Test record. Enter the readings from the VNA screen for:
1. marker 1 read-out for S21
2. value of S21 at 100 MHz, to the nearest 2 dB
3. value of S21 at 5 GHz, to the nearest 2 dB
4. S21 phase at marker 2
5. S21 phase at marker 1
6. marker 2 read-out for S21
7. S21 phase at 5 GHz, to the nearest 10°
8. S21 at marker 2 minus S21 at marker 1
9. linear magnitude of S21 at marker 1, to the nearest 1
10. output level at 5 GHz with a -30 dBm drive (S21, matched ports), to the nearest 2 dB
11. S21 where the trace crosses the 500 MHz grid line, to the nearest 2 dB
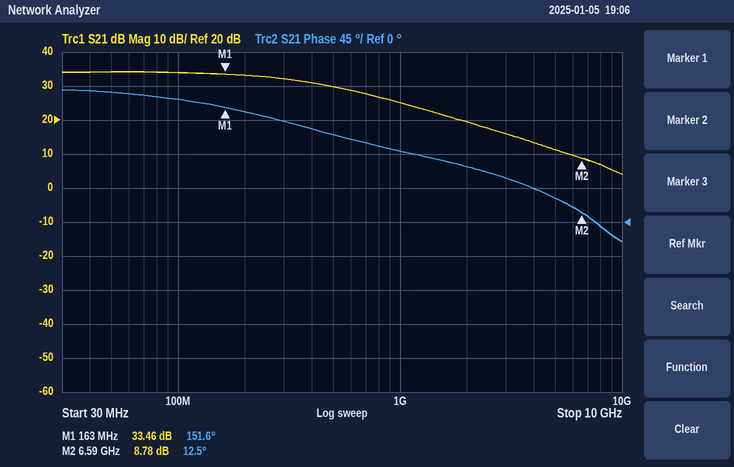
33.46 dB
34 dB
12 dB
12.5°
151.6°
8.78 dB
30°
-24.68 dB
47
-18 dBm
30 dB
